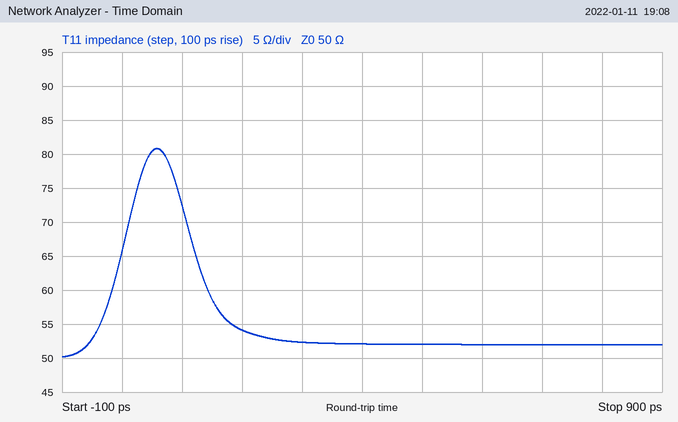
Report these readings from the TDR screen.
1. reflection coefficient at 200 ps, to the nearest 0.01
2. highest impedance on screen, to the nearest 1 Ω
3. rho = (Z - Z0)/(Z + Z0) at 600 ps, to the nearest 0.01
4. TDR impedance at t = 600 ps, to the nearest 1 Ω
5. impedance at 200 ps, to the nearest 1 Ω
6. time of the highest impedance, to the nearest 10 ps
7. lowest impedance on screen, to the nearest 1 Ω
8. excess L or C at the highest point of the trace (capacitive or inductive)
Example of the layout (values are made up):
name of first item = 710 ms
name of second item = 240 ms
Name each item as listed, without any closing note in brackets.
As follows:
reflection coefficient at 200 ps, to the nearest 0.01 = +0.04
highest impedance on screen, to the nearest 1 Ω = 81 Ω
rho = (Z - Z0)/(Z + Z0) at 600 ps, to the nearest 0.01 = +0.02
TDR impedance at t = 600 ps, to the nearest 1 Ω = 52 Ω
impedance at 200 ps, to the nearest 1 Ω = 54 Ω
time of the highest impedance, to the nearest 10 ps = 60 ps
lowest impedance on screen, to the nearest 1 Ω = 50 Ω
excess L or C at the highest point of the trace = inductive
